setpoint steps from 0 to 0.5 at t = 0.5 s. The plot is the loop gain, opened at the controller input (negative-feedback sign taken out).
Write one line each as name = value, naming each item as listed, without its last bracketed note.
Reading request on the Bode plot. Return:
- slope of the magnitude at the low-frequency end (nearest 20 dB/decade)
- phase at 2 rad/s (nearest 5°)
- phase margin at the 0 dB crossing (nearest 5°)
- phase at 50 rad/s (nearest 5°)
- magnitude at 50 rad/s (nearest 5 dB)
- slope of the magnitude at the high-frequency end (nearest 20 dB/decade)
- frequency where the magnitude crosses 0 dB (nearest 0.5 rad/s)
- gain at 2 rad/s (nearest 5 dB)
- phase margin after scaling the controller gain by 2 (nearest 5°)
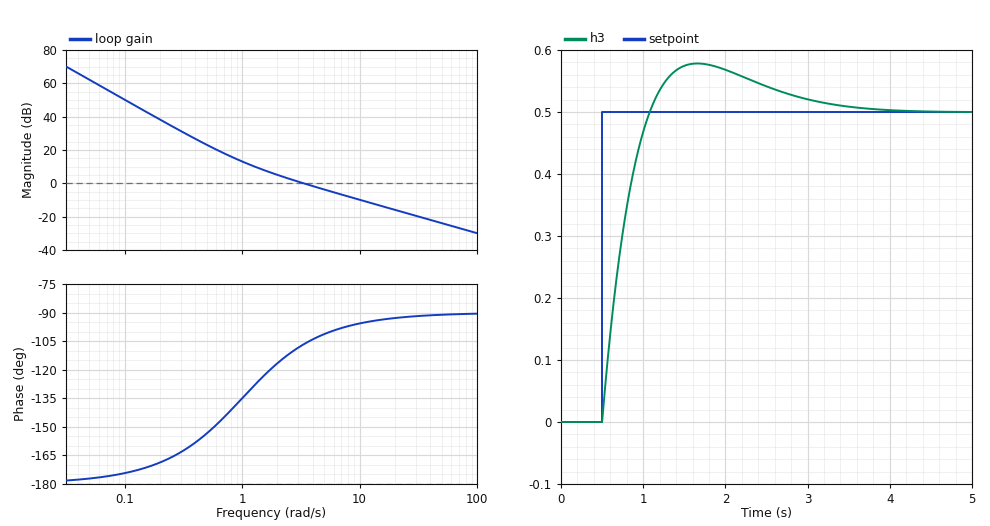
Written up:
slope of the magnitude at the low-frequency end = -40 dB/decade
phase at 2 rad/s = -115°
phase margin at the 0 dB crossing = 75°
phase at 50 rad/s = -90°
magnitude at 50 rad/s = -25 dB
slope of the magnitude at the high-frequency end = -20 dB/decade
frequency where the magnitude crosses 0 dB = 3.5 rad/s
gain at 2 rad/s = 5 dB
phase margin after scaling the controller gain by 2 = 80°
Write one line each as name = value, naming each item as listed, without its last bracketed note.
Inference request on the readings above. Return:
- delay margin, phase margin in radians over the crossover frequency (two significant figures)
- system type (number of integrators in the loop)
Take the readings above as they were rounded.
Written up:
delay margin, phase margin in radians over the crossover frequency = 0.37 s
system type = 2
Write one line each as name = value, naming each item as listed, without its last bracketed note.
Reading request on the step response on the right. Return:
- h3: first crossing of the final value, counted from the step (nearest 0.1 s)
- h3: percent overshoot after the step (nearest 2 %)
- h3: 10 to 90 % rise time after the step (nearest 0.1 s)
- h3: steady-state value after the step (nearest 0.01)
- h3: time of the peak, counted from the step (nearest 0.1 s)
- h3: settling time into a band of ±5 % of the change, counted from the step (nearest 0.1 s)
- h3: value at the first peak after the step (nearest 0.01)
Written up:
h3: first crossing of the final value, counted from the step = 0.6 s
h3: percent overshoot after the step = 16 %
h3: 10 to 90 % rise time after the step = 0.4 s
h3: steady-state value after the step = 0.50
h3: time of the peak, counted from the step = 1.2 s
h3: settling time into a band of ±5 % of the change, counted from the step = 2.4 s
h3: value at the first peak after the step = 0.58
